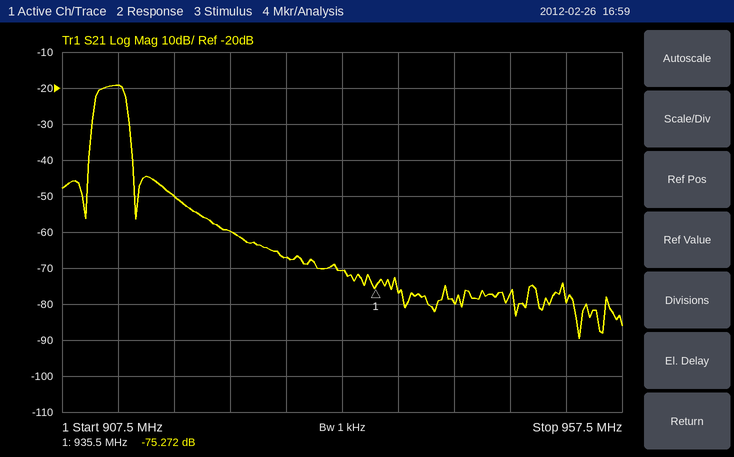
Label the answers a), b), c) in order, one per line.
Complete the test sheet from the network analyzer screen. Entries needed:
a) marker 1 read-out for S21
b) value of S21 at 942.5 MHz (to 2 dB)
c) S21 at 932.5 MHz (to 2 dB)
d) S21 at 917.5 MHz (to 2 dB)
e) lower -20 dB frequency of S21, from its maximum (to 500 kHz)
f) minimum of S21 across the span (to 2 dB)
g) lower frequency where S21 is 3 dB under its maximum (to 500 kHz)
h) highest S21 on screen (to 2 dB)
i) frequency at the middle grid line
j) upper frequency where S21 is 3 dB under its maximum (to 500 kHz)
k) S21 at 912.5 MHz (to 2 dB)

a) -75.272 dB
b) -80 dB
c) -70 dB
d) -50 dB
e) 910.0 MHz
f) -90 dB
g) 910.5 MHz
h) -20 dB
i) 932.5 MHz
j) 913.0 MHz
k) -20 dB
